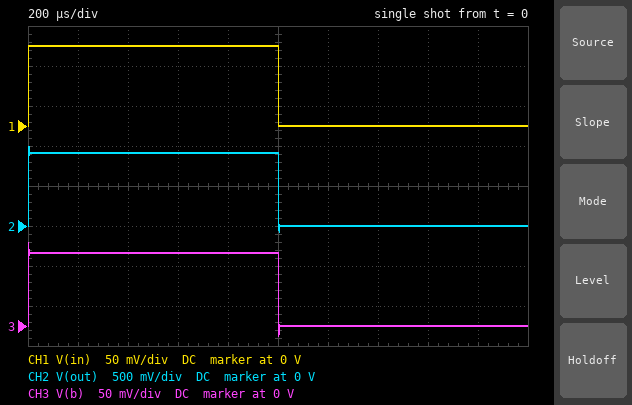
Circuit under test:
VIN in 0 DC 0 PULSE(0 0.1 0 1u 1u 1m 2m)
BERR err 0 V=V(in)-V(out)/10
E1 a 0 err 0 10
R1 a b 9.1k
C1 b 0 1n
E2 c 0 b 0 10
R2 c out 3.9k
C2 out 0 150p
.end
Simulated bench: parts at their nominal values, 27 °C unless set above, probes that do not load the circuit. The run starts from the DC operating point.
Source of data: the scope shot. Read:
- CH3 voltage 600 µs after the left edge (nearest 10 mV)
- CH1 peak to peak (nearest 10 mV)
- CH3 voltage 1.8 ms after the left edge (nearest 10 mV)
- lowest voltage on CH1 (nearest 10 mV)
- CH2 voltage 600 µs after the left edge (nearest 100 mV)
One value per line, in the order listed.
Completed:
90 mV
100 mV
0 V
0 V
900 mV
